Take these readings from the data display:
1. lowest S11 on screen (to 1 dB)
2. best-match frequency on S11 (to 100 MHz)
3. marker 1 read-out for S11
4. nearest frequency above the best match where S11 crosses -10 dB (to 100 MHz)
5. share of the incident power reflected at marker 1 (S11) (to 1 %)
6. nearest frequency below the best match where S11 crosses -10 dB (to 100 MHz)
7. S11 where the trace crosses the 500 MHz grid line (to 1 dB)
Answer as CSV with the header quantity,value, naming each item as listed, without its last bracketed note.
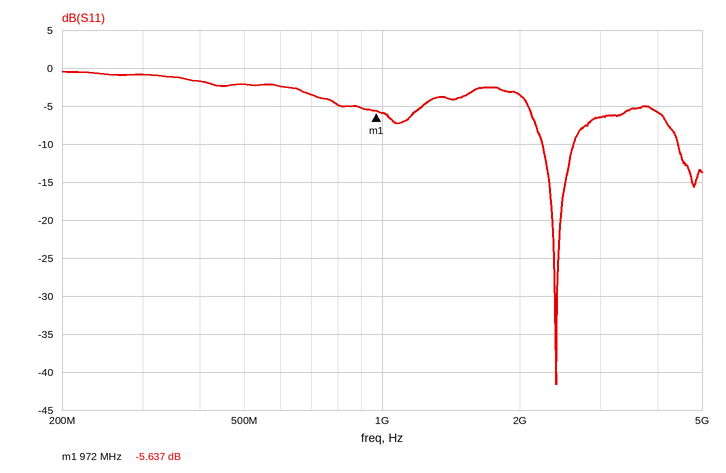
quantity,value
lowest S11 on screen,-42 dB
best-match frequency on S11,2.4 GHz
marker 1 read-out for S11,-5.637 dB
nearest frequency above the best match where S11 crosses -10 dB,2.6 GHz
share of the incident power reflected at marker 1 (S11),27 %
nearest frequency below the best match where S11 crosses -10 dB,2.2 GHz
S11 where the trace crosses the 500 MHz grid line,-2 dB
